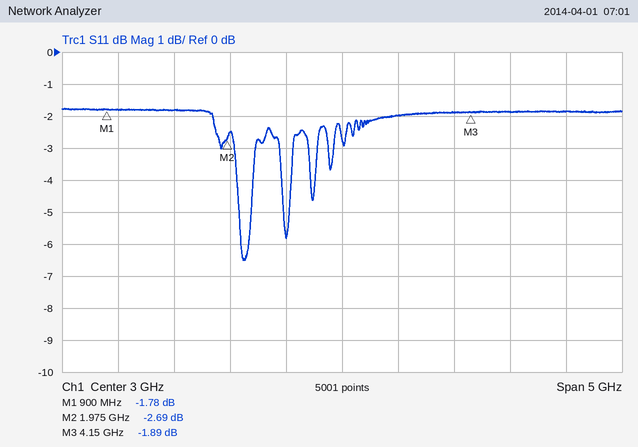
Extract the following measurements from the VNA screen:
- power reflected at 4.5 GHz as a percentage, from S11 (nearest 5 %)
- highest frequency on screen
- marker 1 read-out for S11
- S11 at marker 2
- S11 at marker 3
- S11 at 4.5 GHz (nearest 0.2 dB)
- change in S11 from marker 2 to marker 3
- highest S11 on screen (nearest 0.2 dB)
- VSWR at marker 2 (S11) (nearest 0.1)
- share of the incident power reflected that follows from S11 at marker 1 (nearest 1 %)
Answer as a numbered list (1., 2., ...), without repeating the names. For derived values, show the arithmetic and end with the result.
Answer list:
1. 10^(-1.8/10) ≈ 66.1 %, so 65 % to the nearest 5 %
2. 5.5 GHz
3. -1.78 dB
4. -2.69 dB
5. -1.89 dB
6. -1.8 dB
7. -1.89 − (-2.69) = 0.80 dB
8. -1.8 dB
9. (1 + 0.7337)/(1 − 0.7337) ≈ 6.5
10. 10^(-1.78/10) ≈ 66 %
